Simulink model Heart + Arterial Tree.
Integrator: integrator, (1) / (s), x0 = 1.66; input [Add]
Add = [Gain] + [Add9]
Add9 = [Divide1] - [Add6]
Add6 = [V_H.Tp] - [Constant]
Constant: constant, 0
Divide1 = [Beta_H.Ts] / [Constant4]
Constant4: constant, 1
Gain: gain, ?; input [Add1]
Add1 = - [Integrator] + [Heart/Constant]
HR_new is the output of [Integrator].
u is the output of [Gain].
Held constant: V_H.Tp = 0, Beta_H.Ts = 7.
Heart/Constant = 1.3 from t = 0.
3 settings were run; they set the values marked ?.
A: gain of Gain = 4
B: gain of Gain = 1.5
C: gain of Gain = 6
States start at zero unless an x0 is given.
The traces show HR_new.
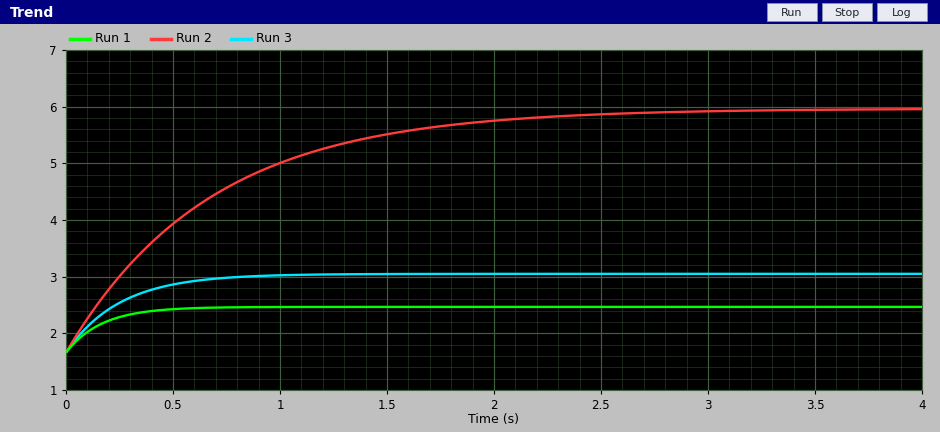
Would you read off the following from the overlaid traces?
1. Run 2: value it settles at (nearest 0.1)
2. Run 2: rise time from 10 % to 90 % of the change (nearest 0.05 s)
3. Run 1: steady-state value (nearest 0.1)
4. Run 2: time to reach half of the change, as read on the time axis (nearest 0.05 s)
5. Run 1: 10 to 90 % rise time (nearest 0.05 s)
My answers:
6.0
1.45 s
2.5
0.45 s
0.35 s
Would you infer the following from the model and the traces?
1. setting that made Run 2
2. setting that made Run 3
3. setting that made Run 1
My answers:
B
A
C
